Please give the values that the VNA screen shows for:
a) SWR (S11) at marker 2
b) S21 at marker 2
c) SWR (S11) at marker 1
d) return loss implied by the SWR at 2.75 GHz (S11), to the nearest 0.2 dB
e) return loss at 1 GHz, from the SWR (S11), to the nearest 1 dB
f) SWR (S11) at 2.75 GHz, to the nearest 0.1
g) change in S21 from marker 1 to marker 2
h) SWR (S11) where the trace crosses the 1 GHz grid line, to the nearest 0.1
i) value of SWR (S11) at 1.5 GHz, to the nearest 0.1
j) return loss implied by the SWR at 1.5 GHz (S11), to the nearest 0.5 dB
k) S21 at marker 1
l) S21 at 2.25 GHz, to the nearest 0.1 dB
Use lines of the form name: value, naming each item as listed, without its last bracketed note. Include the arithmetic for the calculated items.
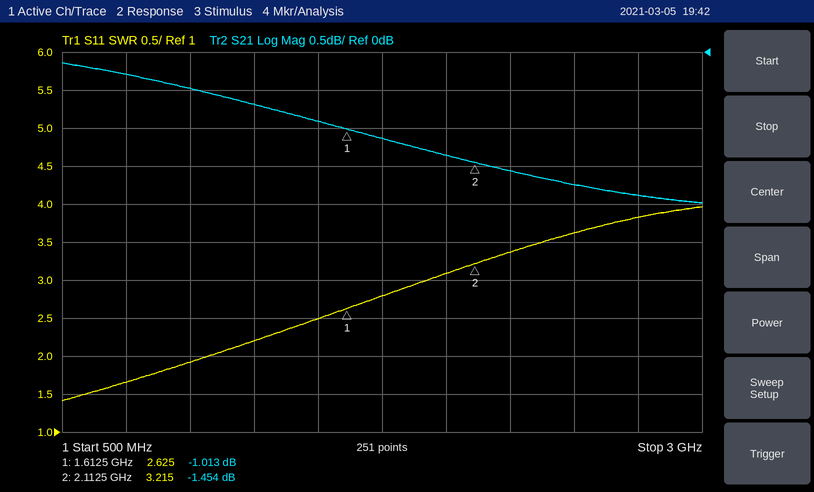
SWR (S11) at marker 2: 3.215
S21 at marker 2: -1.454 dB
SWR (S11) at marker 1: 2.625
return loss implied by the SWR at 2.75 GHz (S11), to the nearest 0.2 dB: −20 log10((3.8 − 1)/(3.8 + 1)) ≈ 4.68 dB, so 4.6 dB to the nearest 0.2 dB
return loss at 1 GHz, from the SWR (S11), to the nearest 1 dB: −20 log10((1.9 − 1)/(1.9 + 1)) ≈ 10 dB
SWR (S11) at 2.75 GHz, to the nearest 0.1: 3.8
change in S21 from marker 1 to marker 2: -1.454 − (-1.013) = -0.441 dB
SWR (S11) where the trace crosses the 1 GHz grid line, to the nearest 0.1: 1.9
value of SWR (S11) at 1.5 GHz, to the nearest 0.1: 2.5
return loss implied by the SWR at 1.5 GHz (S11), to the nearest 0.5 dB: −20 log10((2.5 − 1)/(2.5 + 1)) ≈ 7.36 dB, so 7.5 dB to the nearest 0.5 dB
S21 at marker 1: -1.013 dB
S21 at 2.25 GHz, to the nearest 0.1 dB: -1.6 dB
